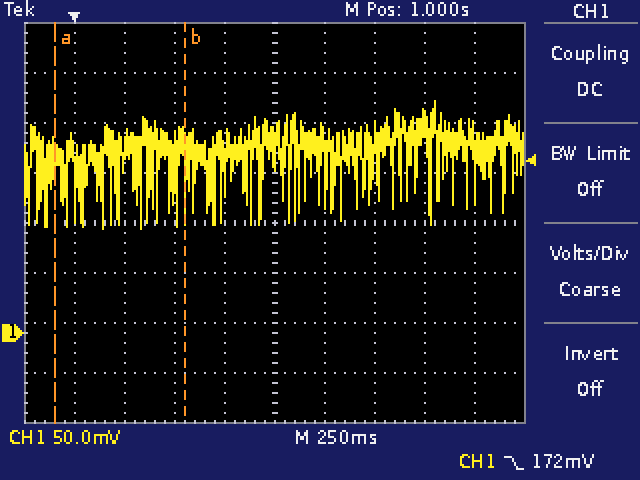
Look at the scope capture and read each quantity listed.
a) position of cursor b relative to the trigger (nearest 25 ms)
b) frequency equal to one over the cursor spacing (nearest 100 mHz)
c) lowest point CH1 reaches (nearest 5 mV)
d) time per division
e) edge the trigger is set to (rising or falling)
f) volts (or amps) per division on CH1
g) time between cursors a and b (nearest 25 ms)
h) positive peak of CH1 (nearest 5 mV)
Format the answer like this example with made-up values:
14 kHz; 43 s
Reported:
+550 ms; 1.5 Hz; 105 mV; 250 ms; falling; 50 mV; 650 ms; 230 mV
